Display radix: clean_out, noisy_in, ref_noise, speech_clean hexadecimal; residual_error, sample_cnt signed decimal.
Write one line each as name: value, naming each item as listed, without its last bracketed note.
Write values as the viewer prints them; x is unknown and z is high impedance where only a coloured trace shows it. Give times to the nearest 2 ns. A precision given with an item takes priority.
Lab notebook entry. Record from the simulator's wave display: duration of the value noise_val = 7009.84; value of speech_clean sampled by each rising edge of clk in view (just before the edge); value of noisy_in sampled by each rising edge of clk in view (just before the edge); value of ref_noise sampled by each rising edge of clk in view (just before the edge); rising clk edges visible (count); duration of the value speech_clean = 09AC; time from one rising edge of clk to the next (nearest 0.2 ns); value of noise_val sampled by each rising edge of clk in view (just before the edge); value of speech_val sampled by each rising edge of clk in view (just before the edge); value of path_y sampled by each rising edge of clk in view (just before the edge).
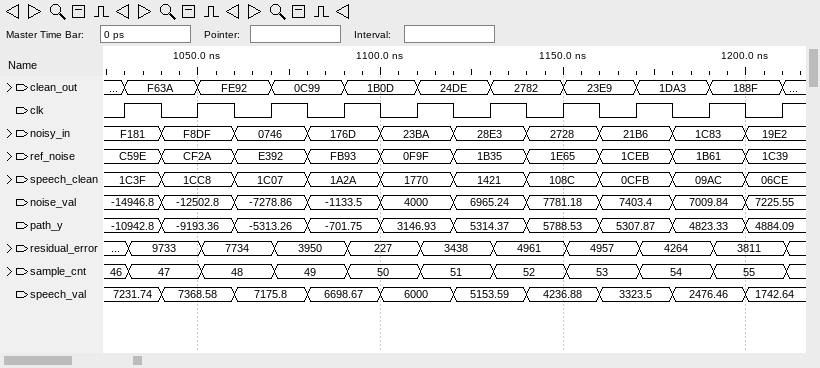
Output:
duration of the value noise_val = 7009.84: 20 ns
value of speech_clean sampled by each rising edge of clk in view: 1C3F, 1CC8, 1C07, 1A2A, 1770, 1421, 108C, 0CFB, 09AC, 06CE
value of noisy_in sampled by each rising edge of clk in view: F181, F8DF, 0746, 176D, 23BA, 28E3, 2728, 21B6, 1C83, 19E2
value of ref_noise sampled by each rising edge of clk in view: C59E, CF2A, E392, FB93, 0F9F, 1B35, 1E65, 1CEB, 1B61, 1C39
rising clk edges visible: 10
duration of the value speech_clean = 09AC: 20 ns
time from one rising edge of clk to the next: 20 ns
value of noise_val sampled by each rising edge of clk in view: -14946.8, -12502.8, -7278.86, -1133.5, 4000, 6965.24, 7781.18, 7403.4, 7009.84, 7225.55
value of speech_val sampled by each rising edge of clk in view: 7231.74, 7368.58, 7175.8, 6698.67, 6000, 5153.59, 4236.88, 3323.5, 2476.46, 1742.64
value of path_y sampled by each rising edge of clk in view: -10942.8, -9193.36, -5313.26, -701.75, 3146.93, 5314.37, 5788.53, 5307.87, 4823.33, 4884.09
